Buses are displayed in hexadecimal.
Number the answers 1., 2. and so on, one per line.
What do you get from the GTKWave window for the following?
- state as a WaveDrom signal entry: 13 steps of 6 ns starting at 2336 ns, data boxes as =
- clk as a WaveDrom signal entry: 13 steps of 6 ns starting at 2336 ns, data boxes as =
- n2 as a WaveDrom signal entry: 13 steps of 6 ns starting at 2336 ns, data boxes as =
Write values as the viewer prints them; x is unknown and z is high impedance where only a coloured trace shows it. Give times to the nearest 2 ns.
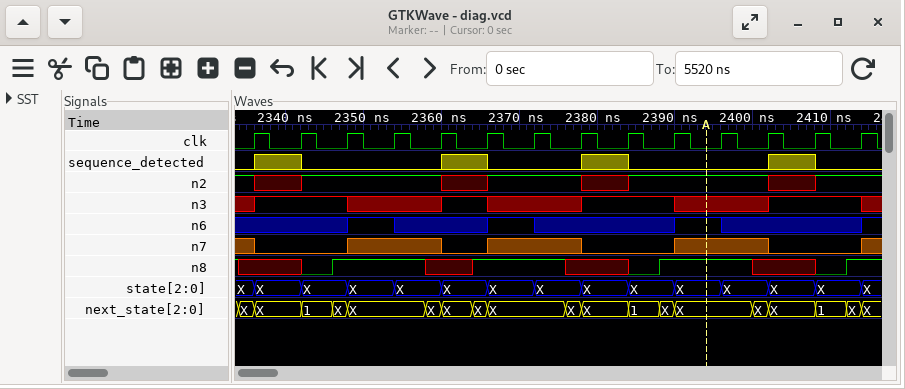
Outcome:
1. {name: 'state', wave: '=============', data: 'X X X X X X X X X X X X X'}
2. {name: 'clk', wave: 'p............'}
3. {name: 'n2', wave: 'x1..x1.x1..x1'}
